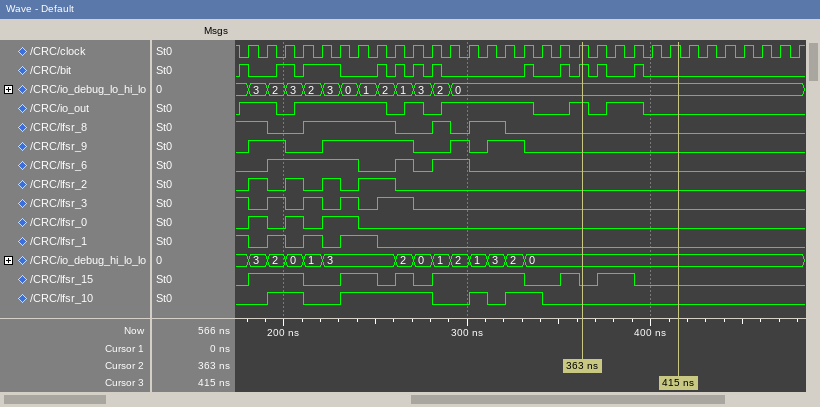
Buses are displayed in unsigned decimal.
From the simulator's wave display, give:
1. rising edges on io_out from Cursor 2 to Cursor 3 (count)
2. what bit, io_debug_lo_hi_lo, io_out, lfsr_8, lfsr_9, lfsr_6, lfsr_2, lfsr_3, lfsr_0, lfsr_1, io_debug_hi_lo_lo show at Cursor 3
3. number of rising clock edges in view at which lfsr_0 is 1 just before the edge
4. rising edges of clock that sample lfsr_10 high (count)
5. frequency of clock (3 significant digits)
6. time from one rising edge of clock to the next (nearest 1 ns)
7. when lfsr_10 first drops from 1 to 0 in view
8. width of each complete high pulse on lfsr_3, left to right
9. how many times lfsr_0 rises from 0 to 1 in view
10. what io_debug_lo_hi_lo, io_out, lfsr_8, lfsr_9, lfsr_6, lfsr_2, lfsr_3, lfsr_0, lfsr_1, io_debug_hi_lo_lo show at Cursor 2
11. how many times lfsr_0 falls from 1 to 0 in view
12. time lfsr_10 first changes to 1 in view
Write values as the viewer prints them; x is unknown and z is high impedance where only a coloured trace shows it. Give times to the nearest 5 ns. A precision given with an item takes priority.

1
bit=0, io_debug_lo_hi_lo=0, io_out=0, lfsr_8=0, lfsr_9=0, lfsr_6=0, lfsr_2=0, lfsr_3=0, lfsr_0=0, lfsr_1=0, io_debug_hi_lo_lo=0
4
10
100 MHz
10 ns
210 ns
10 ns, 10 ns, 10 ns, 20 ns
3
io_debug_lo_hi_lo=0, io_out=1, lfsr_8=0, lfsr_9=0, lfsr_6=0, lfsr_2=0, lfsr_3=0, lfsr_0=0, lfsr_1=0, io_debug_hi_lo_lo=0
3
190 ns
